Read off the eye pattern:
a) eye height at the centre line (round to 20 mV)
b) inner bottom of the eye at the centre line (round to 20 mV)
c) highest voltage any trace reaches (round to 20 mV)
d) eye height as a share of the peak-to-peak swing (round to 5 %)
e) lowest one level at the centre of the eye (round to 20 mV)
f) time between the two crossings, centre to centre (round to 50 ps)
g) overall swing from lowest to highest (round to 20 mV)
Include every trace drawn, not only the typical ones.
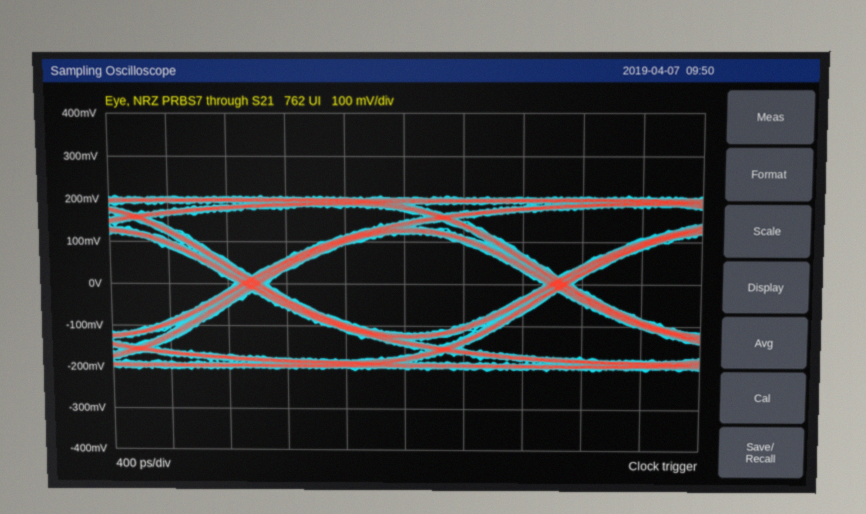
240 mV
-120 mV
200 mV
55 %
120 mV
2.10 ns
420 mV
